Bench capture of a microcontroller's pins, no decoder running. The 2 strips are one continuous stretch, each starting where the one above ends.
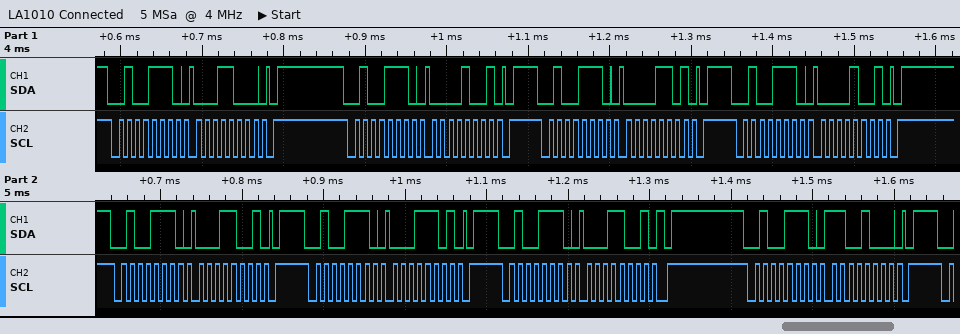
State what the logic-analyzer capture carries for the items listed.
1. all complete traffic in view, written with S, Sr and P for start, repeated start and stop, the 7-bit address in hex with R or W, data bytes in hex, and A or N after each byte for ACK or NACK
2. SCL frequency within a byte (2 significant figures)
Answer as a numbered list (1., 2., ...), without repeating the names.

1. S 27W A 18 A P S 27W A 09 A P S 27W A 0D A P S 27W A 09 A P S 27W A 19 A P S 27W A 1D A P S 27W A 19 A P S 27W A C8 A P
2. 100 kHz
